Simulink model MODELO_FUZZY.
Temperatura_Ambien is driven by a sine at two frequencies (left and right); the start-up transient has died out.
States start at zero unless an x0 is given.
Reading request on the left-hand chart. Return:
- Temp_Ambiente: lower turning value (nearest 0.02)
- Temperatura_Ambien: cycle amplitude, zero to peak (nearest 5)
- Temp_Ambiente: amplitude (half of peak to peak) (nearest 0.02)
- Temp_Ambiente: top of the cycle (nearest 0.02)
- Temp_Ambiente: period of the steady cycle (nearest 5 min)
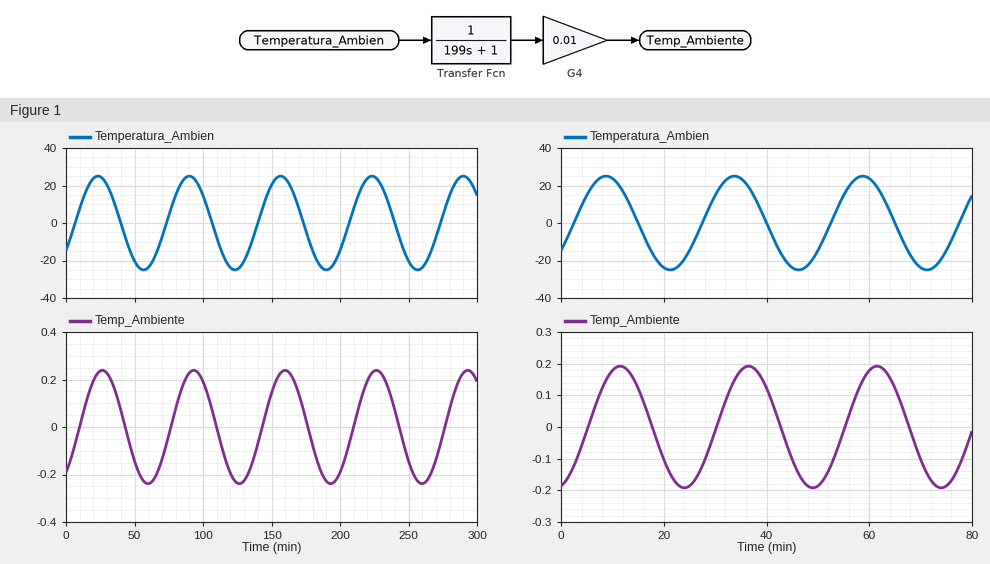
-0.24
25
0.24
0.24
65 min
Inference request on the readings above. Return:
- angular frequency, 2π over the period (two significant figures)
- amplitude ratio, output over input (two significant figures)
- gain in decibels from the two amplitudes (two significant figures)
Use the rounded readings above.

0.097 rad/min
0.0096
-40 dB
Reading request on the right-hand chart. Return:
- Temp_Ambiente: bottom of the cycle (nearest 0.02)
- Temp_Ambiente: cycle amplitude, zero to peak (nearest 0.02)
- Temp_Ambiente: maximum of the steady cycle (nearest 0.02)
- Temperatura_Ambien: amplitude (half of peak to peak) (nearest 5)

-0.20
0.20
0.20
25
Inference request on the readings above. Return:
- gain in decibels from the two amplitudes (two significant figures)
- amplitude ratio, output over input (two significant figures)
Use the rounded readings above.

-42 dB
0.0080
